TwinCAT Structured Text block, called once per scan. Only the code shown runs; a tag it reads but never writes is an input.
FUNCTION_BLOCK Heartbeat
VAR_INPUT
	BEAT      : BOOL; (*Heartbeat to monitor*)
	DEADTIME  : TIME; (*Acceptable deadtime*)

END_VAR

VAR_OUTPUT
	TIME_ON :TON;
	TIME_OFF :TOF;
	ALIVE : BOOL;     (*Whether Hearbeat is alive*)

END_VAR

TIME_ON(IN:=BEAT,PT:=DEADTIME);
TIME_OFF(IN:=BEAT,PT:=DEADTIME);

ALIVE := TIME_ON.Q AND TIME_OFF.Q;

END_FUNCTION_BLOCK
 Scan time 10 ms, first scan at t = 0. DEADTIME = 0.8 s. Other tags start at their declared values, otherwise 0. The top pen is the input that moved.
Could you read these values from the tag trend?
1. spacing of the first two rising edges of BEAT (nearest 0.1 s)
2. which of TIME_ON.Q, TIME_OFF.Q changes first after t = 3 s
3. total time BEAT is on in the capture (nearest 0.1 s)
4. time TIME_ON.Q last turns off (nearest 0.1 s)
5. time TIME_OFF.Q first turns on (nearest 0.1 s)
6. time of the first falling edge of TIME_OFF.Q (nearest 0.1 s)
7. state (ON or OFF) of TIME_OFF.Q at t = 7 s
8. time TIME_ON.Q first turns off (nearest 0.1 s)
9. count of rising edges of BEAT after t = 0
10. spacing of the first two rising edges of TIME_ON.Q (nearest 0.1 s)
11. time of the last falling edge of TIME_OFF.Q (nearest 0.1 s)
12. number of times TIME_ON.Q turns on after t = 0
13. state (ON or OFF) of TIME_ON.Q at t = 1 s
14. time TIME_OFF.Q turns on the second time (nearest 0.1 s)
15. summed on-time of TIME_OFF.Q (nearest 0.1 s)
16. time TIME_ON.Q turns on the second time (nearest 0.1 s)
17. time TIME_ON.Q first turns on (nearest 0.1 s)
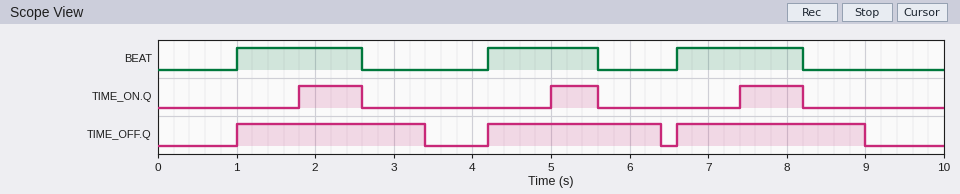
3.2 s
TIME_OFF.Q
4.6 s
8.2 s
1.0 s
3.4 s
ON
2.6 s
3
3.2 s
9.0 s
3
OFF
4.2 s
7.0 s
5.0 s
1.8 s
